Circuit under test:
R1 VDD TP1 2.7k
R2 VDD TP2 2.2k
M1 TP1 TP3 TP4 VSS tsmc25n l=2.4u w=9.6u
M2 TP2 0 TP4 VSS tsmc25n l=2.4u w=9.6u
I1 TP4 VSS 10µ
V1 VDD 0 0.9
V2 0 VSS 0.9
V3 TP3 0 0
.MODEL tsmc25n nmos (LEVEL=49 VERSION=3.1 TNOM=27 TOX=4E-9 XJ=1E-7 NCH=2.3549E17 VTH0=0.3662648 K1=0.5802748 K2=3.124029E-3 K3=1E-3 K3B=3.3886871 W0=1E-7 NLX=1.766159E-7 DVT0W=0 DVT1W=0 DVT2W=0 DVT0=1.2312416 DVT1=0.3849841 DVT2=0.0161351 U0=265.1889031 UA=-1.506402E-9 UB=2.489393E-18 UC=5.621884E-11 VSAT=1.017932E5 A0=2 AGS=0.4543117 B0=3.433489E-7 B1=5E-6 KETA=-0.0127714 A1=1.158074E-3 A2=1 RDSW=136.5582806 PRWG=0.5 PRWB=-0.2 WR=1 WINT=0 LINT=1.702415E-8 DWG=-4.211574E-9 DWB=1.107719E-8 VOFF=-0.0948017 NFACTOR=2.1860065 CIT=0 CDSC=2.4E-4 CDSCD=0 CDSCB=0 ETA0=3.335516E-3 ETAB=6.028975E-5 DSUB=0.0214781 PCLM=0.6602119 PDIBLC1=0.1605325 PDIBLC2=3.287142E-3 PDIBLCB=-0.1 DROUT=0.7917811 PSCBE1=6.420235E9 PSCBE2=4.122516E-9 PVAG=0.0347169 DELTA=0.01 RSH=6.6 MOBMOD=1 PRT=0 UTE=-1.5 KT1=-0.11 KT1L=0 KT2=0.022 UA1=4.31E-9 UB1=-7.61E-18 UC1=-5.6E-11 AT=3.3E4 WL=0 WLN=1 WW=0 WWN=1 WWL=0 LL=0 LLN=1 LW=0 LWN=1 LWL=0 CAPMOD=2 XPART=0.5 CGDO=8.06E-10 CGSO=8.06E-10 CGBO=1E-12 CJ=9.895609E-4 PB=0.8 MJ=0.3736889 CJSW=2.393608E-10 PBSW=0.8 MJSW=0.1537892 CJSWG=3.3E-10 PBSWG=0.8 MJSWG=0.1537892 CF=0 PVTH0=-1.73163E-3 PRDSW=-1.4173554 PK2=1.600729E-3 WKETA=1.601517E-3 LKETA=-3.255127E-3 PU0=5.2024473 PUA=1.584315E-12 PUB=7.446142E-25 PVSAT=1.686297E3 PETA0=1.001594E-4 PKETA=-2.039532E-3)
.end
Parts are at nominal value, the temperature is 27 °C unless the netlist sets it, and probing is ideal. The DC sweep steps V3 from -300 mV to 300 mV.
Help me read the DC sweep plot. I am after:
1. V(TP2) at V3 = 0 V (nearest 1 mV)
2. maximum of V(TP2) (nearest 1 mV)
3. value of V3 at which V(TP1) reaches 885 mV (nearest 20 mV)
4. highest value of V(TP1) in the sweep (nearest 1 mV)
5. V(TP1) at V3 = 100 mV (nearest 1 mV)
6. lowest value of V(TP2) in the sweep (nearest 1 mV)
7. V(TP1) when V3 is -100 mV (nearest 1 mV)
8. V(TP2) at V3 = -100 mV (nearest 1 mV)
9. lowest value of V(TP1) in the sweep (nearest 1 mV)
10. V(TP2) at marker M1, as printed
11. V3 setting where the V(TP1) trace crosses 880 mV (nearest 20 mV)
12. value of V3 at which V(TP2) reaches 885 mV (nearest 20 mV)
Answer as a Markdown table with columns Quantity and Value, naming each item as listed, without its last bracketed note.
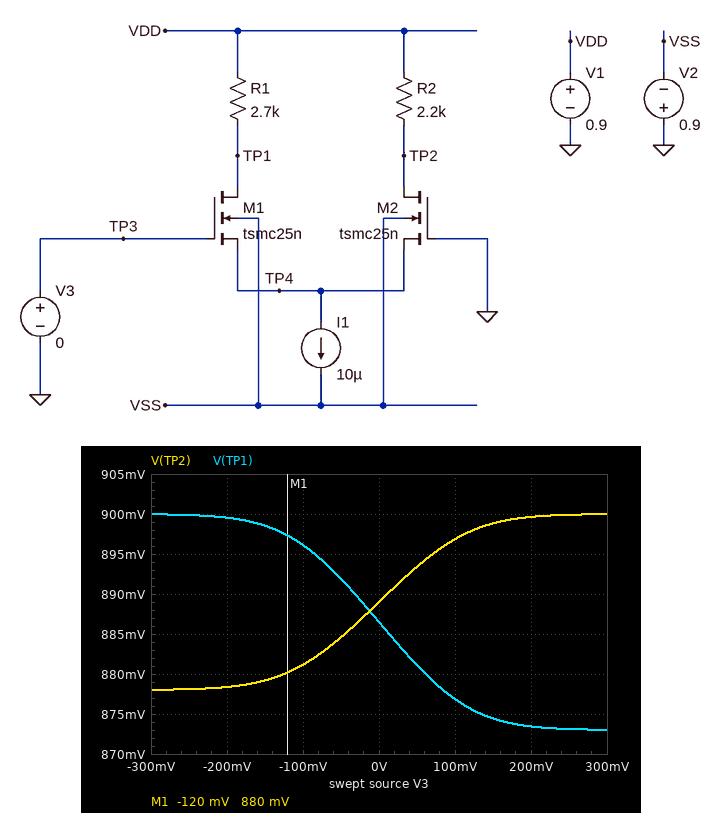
| Quantity | Value |
|---|---|
| V(TP2) at V3 = 0 V | 889 mV |
| maximum of V(TP2) | 900 mV |
| value of V3 at which V(TP1) reaches 885 mV | 20 mV |
| highest value of V(TP1) in the sweep | 900 mV |
| V(TP1) at V3 = 100 mV | 877 mV |
| lowest value of V(TP2) in the sweep | 878 mV |
| V(TP1) when V3 is -100 mV | 896 mV |
| V(TP2) at V3 = -100 mV | 881 mV |
| lowest value of V(TP1) in the sweep | 873 mV |
| V(TP2) at marker M1, as printed | 880 mV |
| V3 setting where the V(TP1) trace crosses 880 mV | 60 mV |
| value of V3 at which V(TP2) reaches 885 mV | -40 mV |
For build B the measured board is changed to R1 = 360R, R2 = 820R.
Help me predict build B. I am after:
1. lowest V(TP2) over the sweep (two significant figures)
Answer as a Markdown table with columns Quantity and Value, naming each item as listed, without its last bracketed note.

| Quantity | Value |
|---|---|
| lowest V(TP2) over the sweep | 890 mV |
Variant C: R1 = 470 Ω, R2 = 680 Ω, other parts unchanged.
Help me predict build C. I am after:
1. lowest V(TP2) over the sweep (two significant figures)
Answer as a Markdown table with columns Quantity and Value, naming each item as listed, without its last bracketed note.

| Quantity | Value |
|---|---|
| lowest V(TP2) over the sweep | 890 mV |
